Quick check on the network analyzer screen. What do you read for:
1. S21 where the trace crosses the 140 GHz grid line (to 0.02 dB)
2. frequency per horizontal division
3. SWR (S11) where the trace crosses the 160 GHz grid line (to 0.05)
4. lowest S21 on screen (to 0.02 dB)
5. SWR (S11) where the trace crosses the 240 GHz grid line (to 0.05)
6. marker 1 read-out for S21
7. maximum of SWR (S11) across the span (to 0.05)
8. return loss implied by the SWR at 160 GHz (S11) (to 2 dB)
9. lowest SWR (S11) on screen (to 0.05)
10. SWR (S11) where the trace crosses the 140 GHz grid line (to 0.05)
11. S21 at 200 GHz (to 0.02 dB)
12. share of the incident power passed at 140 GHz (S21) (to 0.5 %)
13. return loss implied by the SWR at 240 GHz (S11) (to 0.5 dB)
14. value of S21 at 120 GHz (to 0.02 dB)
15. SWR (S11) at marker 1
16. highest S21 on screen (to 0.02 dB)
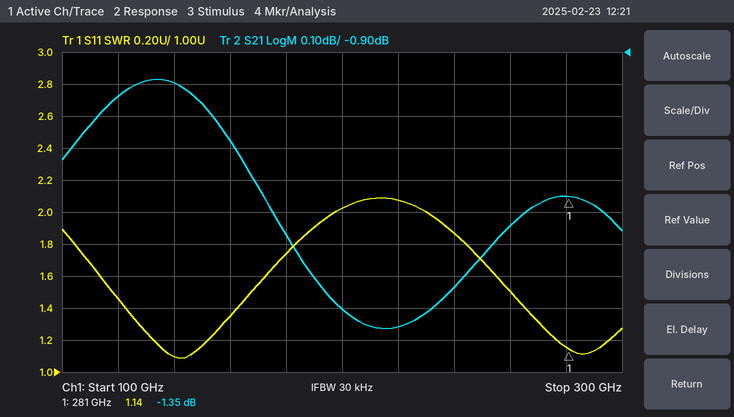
-1.00 dB
20 GHz
1.35
-1.76 dB
1.85
-1.35 dB
2.10
16 dB
1.10
1.10
-1.70 dB
79.5 %
10.5 dB
-1.04 dB
1.14
-0.98 dB
